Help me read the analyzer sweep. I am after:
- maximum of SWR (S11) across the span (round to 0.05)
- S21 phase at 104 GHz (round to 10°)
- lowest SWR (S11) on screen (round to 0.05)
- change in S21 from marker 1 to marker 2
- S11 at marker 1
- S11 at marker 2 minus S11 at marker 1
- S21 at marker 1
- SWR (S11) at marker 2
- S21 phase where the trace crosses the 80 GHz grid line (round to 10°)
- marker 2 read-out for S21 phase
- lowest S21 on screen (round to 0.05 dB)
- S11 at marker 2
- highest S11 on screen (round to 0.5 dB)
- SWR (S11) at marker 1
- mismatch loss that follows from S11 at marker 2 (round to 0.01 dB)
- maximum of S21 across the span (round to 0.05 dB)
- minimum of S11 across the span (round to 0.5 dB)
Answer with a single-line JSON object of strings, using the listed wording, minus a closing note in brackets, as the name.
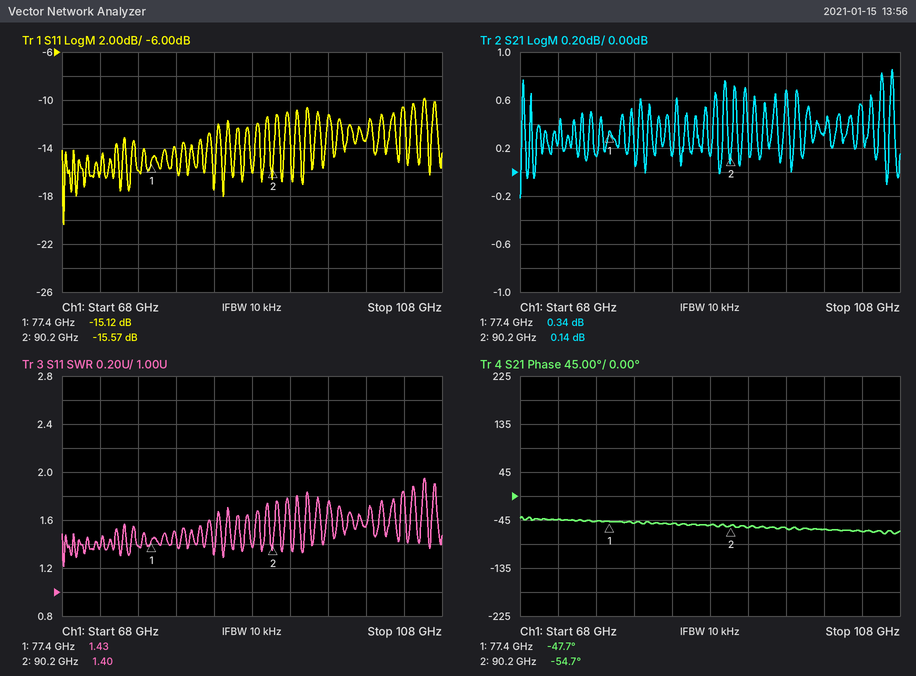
{"maximum of SWR (S11) across the span": "1.95", "S21 phase at 104 GHz": "-70°", "lowest SWR (S11) on screen": "1.20", "change in S21 from marker 1 to marker 2": "-0.20 dB", "S11 at marker 1": "-15.12 dB", "S11 at marker 2 minus S11 at marker 1": "-0.45 dB", "S21 at marker 1": "0.34 dB", "SWR (S11) at marker 2": "1.40", "S21 phase where the trace crosses the 80 GHz grid line": "-50°", "marker 2 read-out for S21 phase": "-54.7°", "lowest S21 on screen": "-0.20 dB", "S11 at marker 2": "-15.57 dB", "highest S11 on screen": "-10.0 dB", "SWR (S11) at marker 1": "1.43", "mismatch loss that follows from S11 at marker 2": "0.12 dB", "maximum of S21 across the span": "0.85 dB", "minimum of S11 across the span": "-20.5 dB"}
